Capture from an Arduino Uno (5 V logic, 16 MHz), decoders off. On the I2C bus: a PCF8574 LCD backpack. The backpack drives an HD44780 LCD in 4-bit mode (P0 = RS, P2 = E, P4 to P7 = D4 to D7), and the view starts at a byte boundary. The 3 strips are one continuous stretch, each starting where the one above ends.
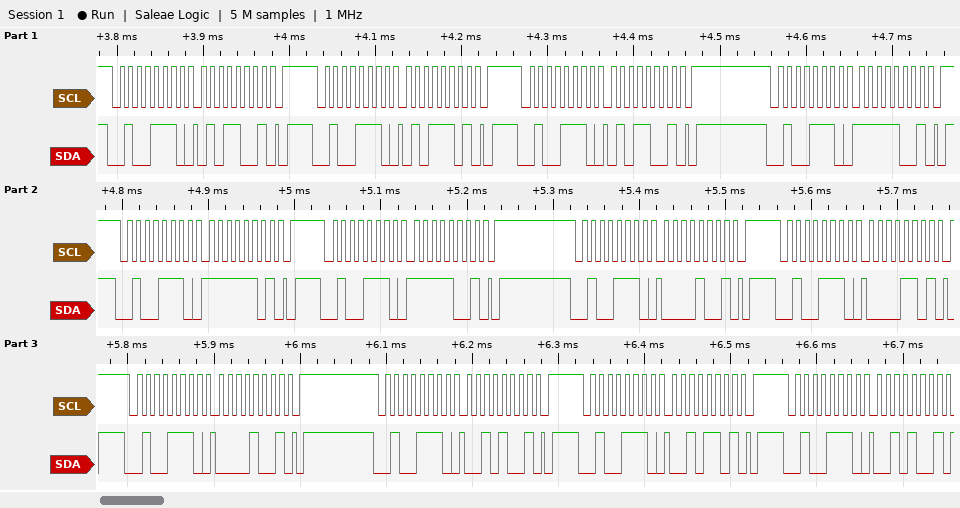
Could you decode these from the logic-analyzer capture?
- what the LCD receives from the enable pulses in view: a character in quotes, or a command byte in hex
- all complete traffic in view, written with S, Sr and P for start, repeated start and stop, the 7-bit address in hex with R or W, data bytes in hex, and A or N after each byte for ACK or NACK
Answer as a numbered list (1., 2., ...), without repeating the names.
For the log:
1. '_' data 0x02
2. S 27W A 59 A P S 27W A 5D A P S 27W A 59 A P S 27W A F9 A P S 27W A FD A P S 27W A F9 A P S 27W A 09 A P S 27W A 0D A P S 27W A 09 A P S 27W A 29 A P S 27W A 2D A P S 27W A 29 A
